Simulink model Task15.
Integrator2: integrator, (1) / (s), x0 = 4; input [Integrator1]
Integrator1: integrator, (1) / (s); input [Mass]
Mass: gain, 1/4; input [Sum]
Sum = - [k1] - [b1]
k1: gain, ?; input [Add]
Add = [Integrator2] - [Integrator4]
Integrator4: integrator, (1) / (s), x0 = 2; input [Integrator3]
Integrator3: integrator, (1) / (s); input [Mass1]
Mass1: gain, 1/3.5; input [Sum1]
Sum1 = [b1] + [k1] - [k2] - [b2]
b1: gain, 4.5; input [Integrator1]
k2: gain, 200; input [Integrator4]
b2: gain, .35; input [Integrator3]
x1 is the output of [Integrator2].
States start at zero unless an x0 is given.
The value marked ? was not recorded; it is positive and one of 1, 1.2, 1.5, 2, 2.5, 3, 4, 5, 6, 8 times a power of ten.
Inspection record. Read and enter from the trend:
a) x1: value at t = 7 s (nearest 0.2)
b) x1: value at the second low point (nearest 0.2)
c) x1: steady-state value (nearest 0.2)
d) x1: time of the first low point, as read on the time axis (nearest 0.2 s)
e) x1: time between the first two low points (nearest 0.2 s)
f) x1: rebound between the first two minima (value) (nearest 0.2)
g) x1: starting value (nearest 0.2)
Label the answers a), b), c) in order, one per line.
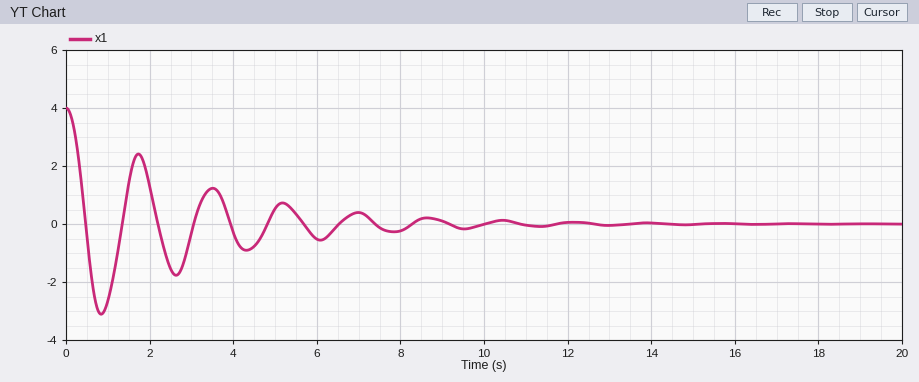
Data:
a) 0.4
b) -1.8
c) 0.0
d) 0.8 s
e) 1.8 s
f) 2.4
g) 4.0
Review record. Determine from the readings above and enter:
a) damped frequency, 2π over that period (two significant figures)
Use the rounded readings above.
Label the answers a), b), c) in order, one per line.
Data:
a) 3.5 rad/s
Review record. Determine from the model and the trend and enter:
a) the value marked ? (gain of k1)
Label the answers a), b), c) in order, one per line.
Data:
a) 80
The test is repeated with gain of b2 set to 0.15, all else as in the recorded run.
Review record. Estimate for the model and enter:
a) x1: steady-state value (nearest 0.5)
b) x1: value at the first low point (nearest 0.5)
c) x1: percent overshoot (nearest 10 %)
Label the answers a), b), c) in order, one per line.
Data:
a) 0.0
b) -3.0
c) 80 %
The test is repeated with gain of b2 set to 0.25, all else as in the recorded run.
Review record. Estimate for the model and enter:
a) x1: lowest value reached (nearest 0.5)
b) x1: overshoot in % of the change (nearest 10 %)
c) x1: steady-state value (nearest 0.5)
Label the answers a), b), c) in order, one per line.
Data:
a) -3.0
b) 80 %
c) 0.0
